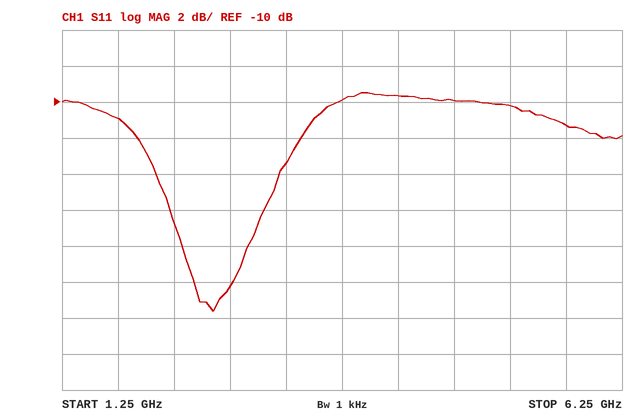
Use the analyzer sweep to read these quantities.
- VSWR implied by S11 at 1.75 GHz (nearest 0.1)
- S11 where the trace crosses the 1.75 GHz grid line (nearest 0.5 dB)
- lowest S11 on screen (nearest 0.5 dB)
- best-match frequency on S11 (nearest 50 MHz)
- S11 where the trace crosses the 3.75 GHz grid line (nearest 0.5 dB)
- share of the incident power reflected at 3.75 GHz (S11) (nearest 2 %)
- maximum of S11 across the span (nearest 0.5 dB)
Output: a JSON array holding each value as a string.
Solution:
["1.8", "-11.0 dB", "-21.5 dB", "2.60 GHz", "-10.0 dB", "10 %", "-9.5 dB"]
